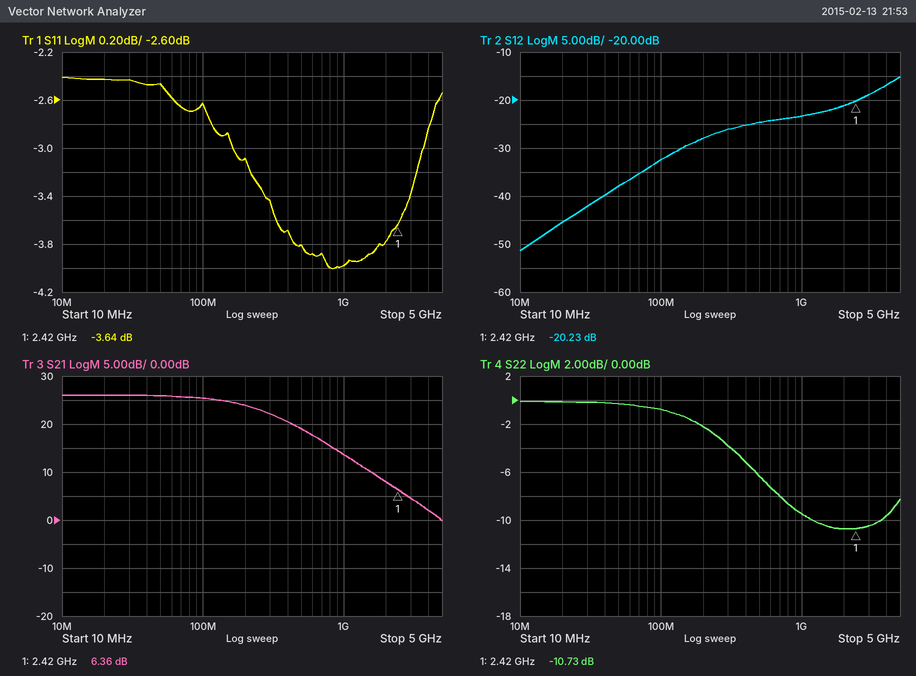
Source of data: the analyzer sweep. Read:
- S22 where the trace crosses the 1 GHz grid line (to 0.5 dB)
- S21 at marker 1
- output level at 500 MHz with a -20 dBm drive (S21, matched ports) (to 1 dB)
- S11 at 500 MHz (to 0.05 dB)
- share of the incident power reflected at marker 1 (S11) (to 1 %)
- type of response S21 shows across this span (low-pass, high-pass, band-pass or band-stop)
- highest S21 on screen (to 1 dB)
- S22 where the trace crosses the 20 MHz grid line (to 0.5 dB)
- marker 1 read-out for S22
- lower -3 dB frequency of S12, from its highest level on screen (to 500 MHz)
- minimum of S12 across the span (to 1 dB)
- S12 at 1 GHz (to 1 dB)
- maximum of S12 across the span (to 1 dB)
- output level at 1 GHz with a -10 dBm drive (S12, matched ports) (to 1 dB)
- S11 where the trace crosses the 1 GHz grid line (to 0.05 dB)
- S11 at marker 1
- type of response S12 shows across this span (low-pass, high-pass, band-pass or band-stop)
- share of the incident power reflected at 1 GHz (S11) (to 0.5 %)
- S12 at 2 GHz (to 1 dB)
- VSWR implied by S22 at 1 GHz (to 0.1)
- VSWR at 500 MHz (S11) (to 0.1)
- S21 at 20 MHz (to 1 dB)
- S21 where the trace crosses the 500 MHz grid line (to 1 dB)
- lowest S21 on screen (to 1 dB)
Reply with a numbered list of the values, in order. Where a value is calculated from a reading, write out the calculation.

1. -9.5 dB
2. 6.36 dB
3. -20 dBm + (19 dB) = -1 dBm
4. -3.80 dB
5. 10^(-3.64/10) ≈ 43 %
6. low-pass
7. 26 dB
8. 0.0 dB
9. -10.73 dB
10. 3.5 GHz
11. -51 dB
12. -23 dB
13. -15 dB
14. -10 dBm + (-23 dB) = -33 dBm
15. -4.00 dB
16. -3.64 dB
17. high-pass
18. 10^(-4/10) ≈ 39.8 %, so 40.0 % to the nearest 0.5 %
19. -21 dB
20. |Γ| = 10^(-9.5/20) = 0.3350; VSWR = (1 + 0.3350)/(1 − 0.3350) ≈ 2.0
21. |Γ| = 10^(-3.8/20) = 0.6457; VSWR = (1 + 0.6457)/(1 − 0.6457) ≈ 4.6
22. 26 dB
23. 19 dB
24. 0 dB
